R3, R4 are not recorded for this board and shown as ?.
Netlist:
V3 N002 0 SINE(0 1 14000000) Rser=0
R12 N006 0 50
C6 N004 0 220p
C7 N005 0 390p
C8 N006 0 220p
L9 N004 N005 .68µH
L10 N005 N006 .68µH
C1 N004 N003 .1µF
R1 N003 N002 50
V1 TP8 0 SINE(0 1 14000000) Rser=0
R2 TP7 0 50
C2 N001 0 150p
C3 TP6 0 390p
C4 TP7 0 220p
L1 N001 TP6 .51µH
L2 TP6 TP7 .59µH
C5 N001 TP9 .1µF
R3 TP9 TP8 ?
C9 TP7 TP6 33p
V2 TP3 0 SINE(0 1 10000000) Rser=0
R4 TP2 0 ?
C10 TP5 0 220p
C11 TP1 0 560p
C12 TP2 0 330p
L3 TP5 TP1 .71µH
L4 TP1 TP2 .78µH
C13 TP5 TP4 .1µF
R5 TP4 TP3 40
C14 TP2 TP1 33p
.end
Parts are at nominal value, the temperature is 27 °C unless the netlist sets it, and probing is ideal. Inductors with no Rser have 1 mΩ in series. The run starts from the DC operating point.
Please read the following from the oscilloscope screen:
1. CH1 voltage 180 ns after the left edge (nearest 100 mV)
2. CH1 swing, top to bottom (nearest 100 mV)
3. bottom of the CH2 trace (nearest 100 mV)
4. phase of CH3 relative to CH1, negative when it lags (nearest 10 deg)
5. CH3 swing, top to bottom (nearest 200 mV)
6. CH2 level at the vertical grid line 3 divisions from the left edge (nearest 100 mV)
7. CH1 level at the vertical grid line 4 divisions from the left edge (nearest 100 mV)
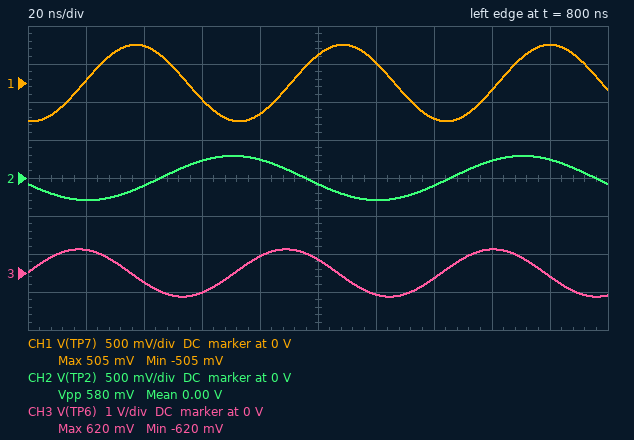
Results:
500 mV
1.0 V
-300 mV
100 deg
1.2 V
200 mV
-400 mV
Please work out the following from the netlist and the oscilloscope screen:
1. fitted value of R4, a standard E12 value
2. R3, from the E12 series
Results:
18 Ω
47 Ω
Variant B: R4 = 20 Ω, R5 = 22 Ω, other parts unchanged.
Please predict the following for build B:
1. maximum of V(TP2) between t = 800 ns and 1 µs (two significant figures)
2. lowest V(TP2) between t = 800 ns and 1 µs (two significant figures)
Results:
450 mV
-450 mV
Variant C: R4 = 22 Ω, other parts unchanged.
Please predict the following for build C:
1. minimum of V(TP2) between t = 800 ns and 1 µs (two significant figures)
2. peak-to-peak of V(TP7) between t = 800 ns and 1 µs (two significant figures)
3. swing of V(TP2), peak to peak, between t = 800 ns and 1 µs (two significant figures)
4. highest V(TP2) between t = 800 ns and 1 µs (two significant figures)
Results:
-340 mV
1.0 V
670 mV
340 mV
